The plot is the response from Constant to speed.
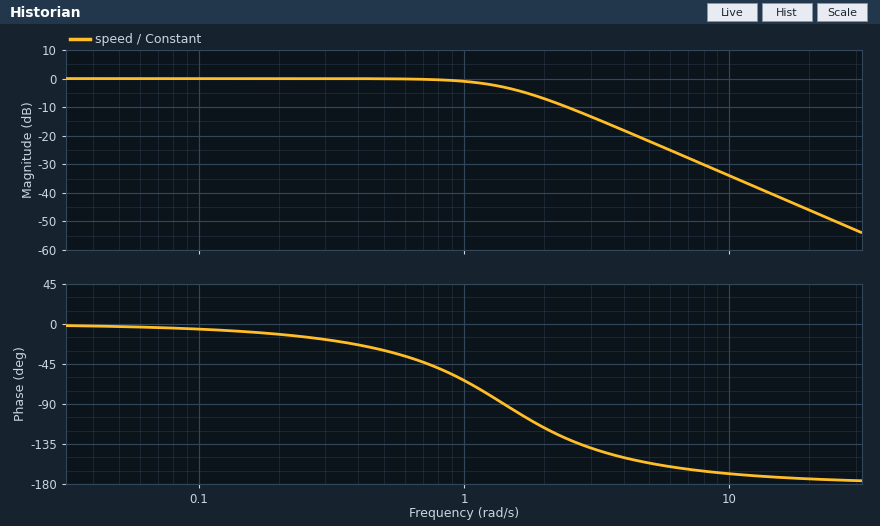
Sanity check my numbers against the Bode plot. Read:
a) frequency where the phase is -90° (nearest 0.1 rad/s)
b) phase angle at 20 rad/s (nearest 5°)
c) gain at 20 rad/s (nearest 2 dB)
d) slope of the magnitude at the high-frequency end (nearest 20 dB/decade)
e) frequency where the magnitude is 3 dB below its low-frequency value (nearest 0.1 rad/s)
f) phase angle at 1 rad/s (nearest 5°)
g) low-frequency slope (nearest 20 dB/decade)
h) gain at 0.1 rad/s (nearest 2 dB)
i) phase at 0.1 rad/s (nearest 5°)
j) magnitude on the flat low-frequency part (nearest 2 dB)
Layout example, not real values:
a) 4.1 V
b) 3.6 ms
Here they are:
a) 1.4 rad/s
b) -175°
c) -46 dB
d) -40 dB/decade
e) 1.4 rad/s
f) -65°
g) 0 dB/decade
h) 0 dB
i) -5°
j) 0 dB
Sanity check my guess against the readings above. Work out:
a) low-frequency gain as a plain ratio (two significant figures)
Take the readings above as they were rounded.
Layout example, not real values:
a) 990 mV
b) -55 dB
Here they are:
a) 1.0
